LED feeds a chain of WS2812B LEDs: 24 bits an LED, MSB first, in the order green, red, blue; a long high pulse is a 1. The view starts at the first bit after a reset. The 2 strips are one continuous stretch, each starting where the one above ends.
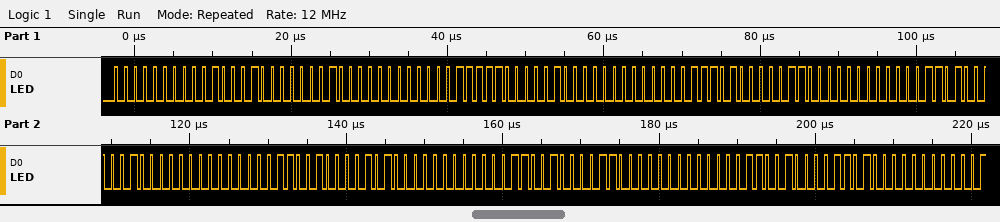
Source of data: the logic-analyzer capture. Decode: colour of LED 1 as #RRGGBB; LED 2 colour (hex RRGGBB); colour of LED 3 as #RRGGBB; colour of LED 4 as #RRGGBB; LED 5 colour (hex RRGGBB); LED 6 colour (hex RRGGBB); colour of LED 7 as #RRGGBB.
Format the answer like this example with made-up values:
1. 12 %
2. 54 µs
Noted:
1. #220002
2. #1F0004
3. #1D0006
4. #1A0008
5. #19000A
6. #19000C
7. #19000D
